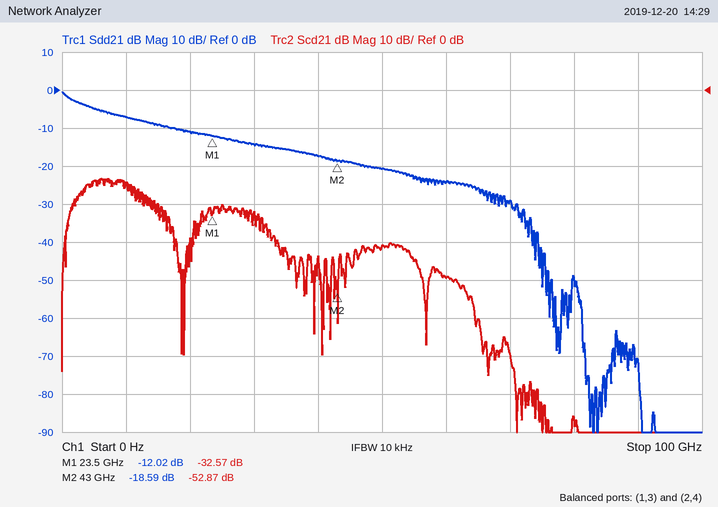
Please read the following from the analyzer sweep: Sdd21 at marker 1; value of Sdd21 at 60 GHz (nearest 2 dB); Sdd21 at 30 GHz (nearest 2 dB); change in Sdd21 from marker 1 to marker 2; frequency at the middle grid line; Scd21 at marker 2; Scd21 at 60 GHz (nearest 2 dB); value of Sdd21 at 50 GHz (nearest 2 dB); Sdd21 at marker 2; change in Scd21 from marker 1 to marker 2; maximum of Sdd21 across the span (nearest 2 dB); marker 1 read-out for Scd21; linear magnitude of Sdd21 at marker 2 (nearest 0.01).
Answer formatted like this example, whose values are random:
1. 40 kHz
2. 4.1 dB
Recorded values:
1. -12.02 dB
2. -24 dB
3. -14 dB
4. -6.57 dB
5. 50 GHz
6. -52.87 dB
7. -50 dB
8. -20 dB
9. -18.59 dB
10. -20.30 dB
11. 0 dB
12. -32.57 dB
13. 0.12
